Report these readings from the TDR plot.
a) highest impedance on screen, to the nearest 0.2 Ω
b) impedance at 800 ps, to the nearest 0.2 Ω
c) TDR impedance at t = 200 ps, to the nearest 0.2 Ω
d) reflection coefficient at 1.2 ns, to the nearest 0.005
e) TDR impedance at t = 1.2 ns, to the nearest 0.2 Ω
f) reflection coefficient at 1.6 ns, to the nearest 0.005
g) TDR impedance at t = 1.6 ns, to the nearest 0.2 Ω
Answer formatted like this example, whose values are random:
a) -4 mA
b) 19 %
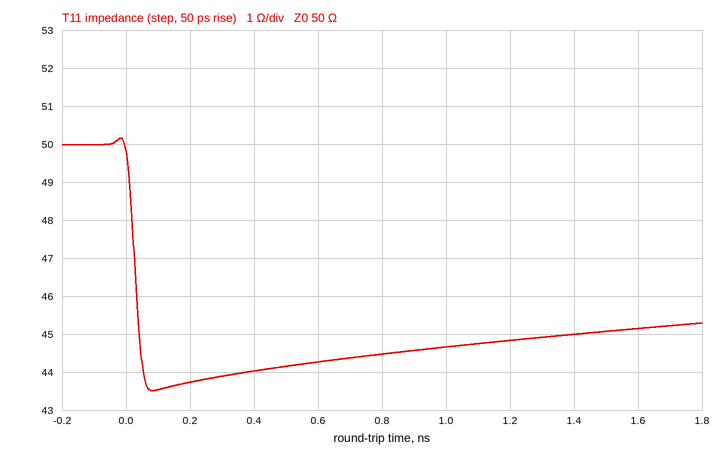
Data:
a) 50.2 Ω
b) 44.4 Ω
c) 43.8 Ω
d) -0.055
e) 44.8 Ω
f) -0.050
g) 45.2 Ω
